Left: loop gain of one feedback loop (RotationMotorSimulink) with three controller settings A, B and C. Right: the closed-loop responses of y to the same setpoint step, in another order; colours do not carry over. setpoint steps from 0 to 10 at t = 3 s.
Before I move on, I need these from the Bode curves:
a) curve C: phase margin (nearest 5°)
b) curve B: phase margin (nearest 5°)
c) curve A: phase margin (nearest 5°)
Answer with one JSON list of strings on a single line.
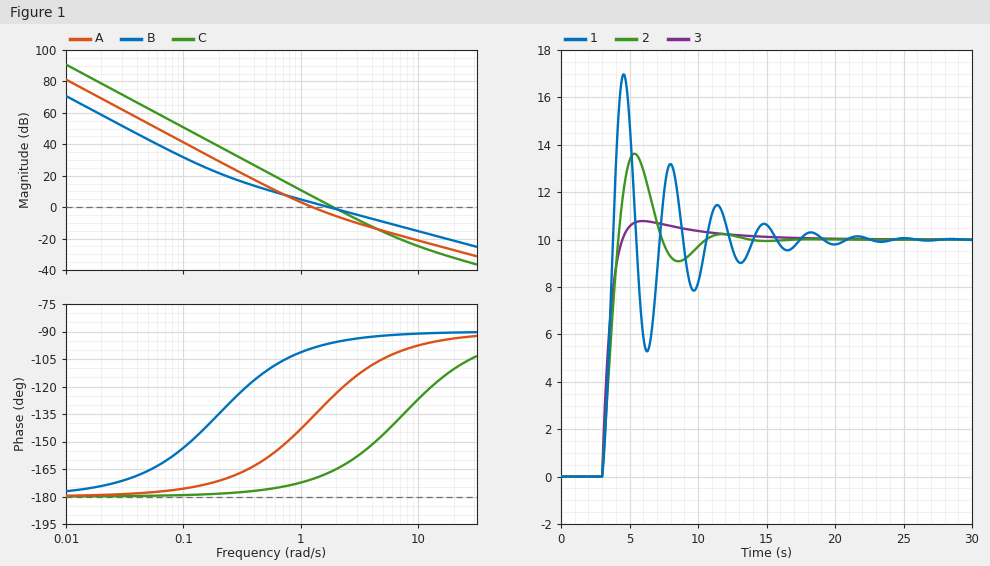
["15°", "85°", "45°"]
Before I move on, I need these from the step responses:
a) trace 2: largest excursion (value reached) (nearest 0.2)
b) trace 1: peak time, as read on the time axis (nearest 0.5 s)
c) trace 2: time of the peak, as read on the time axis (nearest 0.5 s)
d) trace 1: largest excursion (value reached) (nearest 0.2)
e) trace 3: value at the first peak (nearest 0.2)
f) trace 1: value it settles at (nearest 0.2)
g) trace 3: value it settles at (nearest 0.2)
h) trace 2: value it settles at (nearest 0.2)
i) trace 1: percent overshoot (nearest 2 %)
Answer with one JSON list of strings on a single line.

["13.6", "4.5 s", "5.5 s", "17.0", "10.8", "10.0", "10.0", "10.0", "70 %"]
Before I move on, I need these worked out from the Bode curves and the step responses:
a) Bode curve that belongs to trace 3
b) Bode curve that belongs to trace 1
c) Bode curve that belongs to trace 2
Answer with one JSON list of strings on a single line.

["B", "C", "A"]
